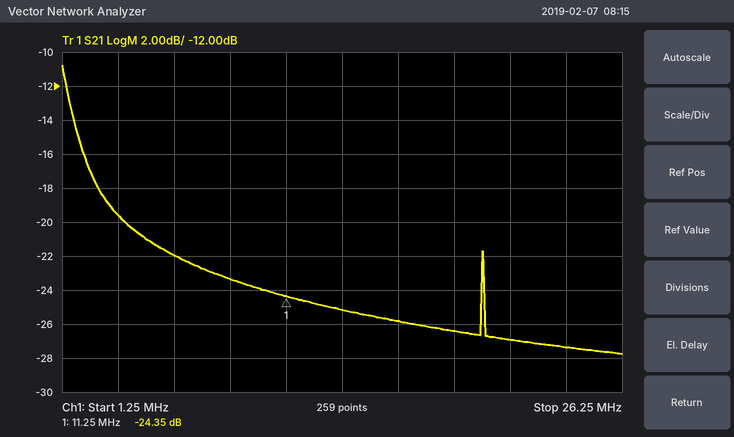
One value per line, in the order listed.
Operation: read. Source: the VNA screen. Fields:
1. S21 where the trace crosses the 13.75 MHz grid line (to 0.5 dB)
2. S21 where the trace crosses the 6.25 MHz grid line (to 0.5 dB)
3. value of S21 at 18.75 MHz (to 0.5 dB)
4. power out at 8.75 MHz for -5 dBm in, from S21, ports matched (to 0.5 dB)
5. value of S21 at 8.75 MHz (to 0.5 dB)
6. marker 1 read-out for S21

-25.0 dB
-22.0 dB
-26.5 dB
-28.5 dBm
-23.5 dB
-24.35 dB
